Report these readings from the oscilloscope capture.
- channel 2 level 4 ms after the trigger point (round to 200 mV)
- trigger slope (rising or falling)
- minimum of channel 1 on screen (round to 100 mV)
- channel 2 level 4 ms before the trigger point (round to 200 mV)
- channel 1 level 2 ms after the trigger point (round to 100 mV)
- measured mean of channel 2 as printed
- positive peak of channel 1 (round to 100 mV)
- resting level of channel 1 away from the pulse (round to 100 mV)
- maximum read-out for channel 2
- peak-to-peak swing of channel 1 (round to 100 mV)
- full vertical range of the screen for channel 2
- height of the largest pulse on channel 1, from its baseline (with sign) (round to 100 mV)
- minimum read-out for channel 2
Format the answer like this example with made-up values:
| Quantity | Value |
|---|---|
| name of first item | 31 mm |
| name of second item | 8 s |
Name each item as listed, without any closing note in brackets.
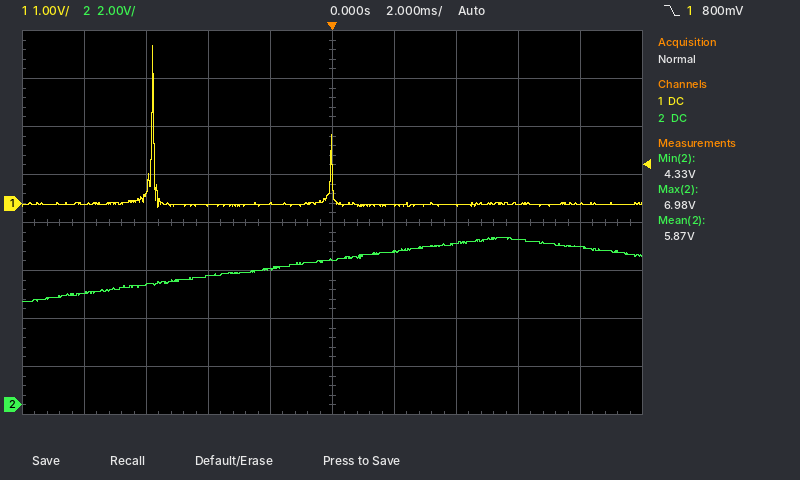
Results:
| Quantity | Value |
|---|---|
| channel 2 level 4 ms after the trigger point | 6.8 V |
| trigger slope | falling |
| minimum of channel 1 on screen | -100 mV |
| channel 2 level 4 ms before the trigger point | 5.4 V |
| channel 1 level 2 ms after the trigger point | 0.0 V |
| measured mean of channel 2 as printed | 5.87 V |
| positive peak of channel 1 | 3.3 V |
| resting level of channel 1 away from the pulse | 0.0 V |
| maximum read-out for channel 2 | 6.98 V |
| peak-to-peak swing of channel 1 | 3.4 V |
| full vertical range of the screen for channel 2 | 16 V |
| height of the largest pulse on channel 1, from its baseline (with sign) | +3.3 V |
| minimum read-out for channel 2 | 4.33 V |
